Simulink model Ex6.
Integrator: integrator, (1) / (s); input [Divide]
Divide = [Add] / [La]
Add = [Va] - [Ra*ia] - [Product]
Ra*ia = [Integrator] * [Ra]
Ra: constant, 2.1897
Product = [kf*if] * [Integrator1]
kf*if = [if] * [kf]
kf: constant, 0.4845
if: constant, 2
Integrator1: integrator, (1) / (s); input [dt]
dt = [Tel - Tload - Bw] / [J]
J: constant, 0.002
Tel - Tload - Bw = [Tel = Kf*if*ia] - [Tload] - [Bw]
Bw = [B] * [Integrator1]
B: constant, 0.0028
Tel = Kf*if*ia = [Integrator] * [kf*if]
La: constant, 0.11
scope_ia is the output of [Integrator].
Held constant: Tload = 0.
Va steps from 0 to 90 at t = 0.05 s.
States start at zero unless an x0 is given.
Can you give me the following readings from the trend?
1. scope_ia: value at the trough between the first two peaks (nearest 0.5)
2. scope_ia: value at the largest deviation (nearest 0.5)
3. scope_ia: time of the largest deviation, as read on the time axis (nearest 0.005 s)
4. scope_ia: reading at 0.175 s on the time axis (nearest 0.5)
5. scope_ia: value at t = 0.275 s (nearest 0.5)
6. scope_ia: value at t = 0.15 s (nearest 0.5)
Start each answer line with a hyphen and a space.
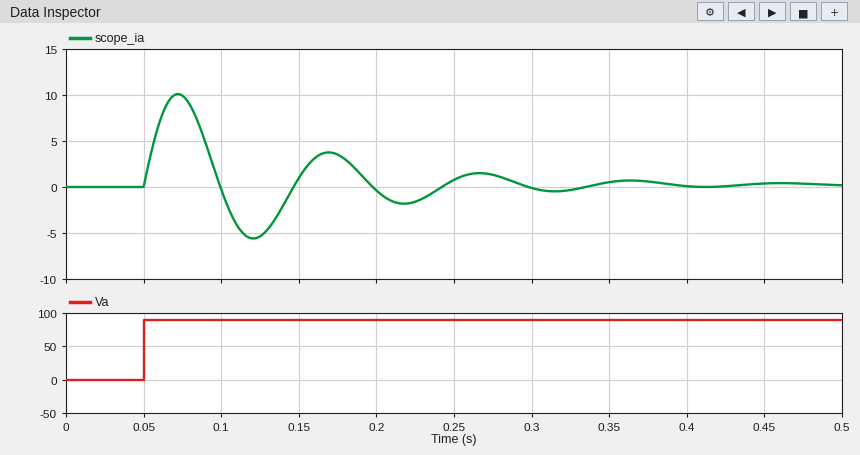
- -5.5
- 10.0
- 0.070 s
- 3.5
- 1.5
- 1.0
